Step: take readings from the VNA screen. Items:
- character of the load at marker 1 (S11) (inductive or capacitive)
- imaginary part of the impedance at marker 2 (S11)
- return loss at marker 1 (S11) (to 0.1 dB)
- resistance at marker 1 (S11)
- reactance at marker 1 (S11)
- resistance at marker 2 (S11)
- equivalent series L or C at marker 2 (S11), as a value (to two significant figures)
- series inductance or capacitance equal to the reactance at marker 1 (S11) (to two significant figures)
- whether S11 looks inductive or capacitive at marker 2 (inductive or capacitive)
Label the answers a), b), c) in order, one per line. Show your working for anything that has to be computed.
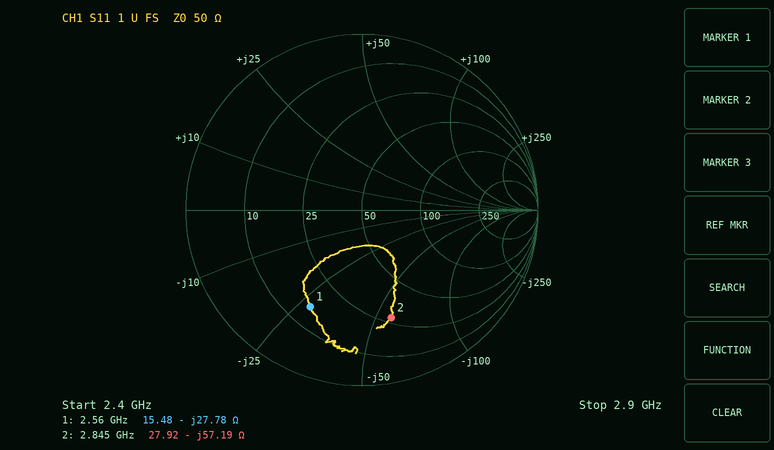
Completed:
a) capacitive
b) -57.19 Ω
c) 4.1 dB
d) 15.48 Ω
e) -27.78 Ω
f) 27.92 Ω
g) C = 1/(2π × 2.845 GHz × 57.19 Ω) ≈ 978 fF, so 980 fF to two significant figures
h) C = 1/(2π × 2.56 GHz × 27.78 Ω) ≈ 2.2 pF
i) capacitive
